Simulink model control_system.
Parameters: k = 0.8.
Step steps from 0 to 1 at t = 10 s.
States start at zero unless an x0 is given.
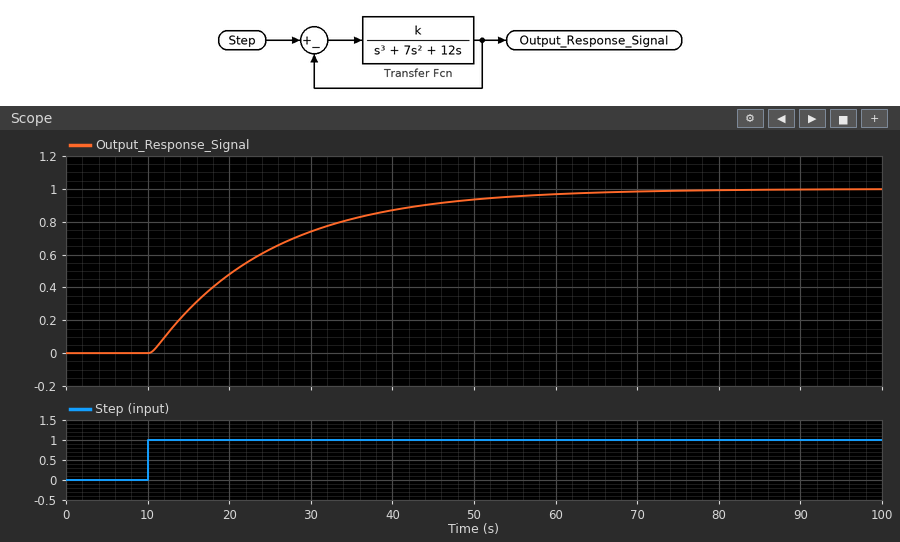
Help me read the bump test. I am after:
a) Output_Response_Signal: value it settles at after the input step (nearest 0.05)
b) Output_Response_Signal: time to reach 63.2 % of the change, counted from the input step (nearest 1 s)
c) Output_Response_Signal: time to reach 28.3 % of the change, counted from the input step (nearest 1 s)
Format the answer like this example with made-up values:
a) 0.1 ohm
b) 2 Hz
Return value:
a) 1.00
b) 15 s
c) 5 s
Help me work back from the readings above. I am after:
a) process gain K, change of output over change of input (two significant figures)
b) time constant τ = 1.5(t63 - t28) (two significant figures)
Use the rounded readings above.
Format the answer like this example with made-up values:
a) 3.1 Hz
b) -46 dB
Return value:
a) 1.0
b) 15 s
